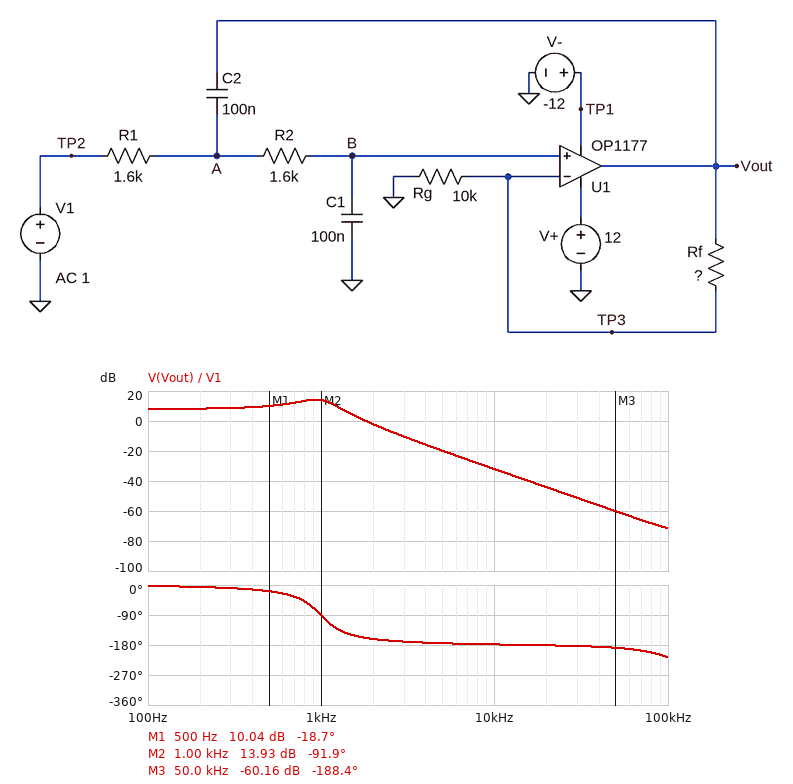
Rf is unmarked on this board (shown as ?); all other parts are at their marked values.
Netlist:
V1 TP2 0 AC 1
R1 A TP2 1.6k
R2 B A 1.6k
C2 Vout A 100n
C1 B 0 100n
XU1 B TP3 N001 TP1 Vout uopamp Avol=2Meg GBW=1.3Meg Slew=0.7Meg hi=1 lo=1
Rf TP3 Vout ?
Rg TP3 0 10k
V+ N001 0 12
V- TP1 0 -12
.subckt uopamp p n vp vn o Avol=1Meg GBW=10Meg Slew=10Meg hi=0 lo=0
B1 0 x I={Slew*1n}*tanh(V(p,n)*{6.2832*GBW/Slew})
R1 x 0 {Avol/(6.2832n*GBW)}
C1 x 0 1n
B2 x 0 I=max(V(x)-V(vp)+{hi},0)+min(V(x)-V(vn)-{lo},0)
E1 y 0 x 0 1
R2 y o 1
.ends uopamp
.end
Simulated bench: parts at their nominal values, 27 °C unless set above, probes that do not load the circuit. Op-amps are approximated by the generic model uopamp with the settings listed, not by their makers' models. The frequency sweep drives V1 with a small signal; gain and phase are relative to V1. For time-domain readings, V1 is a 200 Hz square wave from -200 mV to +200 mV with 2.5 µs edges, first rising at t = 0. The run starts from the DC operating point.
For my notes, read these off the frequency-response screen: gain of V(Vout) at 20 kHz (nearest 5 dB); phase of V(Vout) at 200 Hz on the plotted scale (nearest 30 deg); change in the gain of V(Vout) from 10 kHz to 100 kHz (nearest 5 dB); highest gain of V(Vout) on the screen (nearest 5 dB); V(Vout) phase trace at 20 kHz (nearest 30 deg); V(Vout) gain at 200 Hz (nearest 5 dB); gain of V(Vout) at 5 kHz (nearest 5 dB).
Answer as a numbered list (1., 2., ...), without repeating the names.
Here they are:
1. -45 dB
2. 0 deg
3. -40 dB
4. 15 dB
5. -180 deg
6. 10 dB
7. -20 dB
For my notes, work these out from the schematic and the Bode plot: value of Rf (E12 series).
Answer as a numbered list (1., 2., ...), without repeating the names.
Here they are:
1. 15 kΩ
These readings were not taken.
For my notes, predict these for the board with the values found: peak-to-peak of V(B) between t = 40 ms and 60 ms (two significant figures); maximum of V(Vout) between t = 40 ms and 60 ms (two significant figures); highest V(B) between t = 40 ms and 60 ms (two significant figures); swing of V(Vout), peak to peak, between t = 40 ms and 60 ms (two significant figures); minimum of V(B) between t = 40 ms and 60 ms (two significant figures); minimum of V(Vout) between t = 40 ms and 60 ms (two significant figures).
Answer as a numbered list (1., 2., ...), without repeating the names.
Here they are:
1. 760 mV
2. 950 mV
3. 380 mV
4. 1.9 V
5. -380 mV
6. -950 mV
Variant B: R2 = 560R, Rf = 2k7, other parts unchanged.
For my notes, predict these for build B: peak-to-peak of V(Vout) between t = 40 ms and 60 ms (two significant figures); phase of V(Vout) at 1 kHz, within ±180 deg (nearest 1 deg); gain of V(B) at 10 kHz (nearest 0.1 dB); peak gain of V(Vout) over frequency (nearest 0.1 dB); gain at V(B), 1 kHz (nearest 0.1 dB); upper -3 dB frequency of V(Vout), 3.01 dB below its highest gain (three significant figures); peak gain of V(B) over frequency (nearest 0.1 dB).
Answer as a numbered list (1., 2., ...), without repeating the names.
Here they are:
1. 510 mV
2. -59 deg
3. -31.2 dB
4. 2.1 dB
5. -2.0 dB
6. 1.23 kHz
7. 0 dB
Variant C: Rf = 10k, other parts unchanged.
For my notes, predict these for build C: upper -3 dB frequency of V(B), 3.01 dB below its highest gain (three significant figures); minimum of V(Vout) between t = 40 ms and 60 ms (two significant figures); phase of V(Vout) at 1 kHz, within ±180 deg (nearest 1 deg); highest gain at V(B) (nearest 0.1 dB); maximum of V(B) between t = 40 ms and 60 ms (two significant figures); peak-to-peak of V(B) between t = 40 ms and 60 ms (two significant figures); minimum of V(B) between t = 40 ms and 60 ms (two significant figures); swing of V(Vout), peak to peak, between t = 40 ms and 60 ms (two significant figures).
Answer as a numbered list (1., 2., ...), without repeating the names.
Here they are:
1. 1.16 kHz
2. -530 mV
3. -91 deg
4. 1.3 dB
5. 270 mV
6. 530 mV
7. -270 mV
8. 1.1 V
